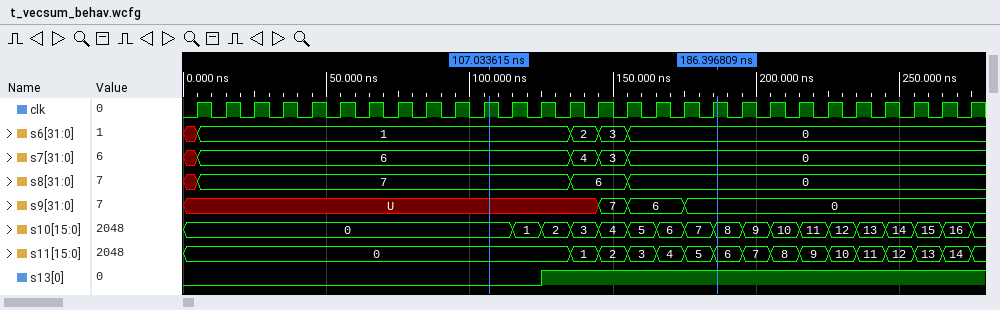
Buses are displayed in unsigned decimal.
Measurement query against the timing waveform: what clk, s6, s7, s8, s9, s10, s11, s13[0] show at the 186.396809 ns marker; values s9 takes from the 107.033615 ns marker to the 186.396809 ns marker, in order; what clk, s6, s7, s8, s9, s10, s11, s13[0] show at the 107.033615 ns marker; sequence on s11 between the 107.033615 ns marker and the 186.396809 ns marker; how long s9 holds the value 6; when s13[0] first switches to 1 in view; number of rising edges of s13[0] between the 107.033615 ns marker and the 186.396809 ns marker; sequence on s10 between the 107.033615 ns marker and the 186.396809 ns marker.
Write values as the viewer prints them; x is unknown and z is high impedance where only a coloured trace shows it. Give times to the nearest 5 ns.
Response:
clk=1, s6=0, s7=0, s8=0, s9=0, s10=8, s11=6, s13[0]=1
U, 7, 6, 0
clk=1, s6=1, s7=6, s8=7, s9=U, s10=0, s11=0, s13[0]=0
0, 1, 2, 3, 4, 5, 6
20 ns
125 ns
1
0, 1, 2, 3, 4, 5, 6, 7, 8
